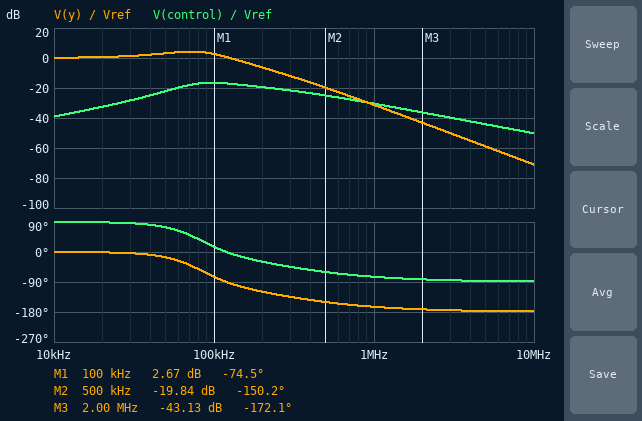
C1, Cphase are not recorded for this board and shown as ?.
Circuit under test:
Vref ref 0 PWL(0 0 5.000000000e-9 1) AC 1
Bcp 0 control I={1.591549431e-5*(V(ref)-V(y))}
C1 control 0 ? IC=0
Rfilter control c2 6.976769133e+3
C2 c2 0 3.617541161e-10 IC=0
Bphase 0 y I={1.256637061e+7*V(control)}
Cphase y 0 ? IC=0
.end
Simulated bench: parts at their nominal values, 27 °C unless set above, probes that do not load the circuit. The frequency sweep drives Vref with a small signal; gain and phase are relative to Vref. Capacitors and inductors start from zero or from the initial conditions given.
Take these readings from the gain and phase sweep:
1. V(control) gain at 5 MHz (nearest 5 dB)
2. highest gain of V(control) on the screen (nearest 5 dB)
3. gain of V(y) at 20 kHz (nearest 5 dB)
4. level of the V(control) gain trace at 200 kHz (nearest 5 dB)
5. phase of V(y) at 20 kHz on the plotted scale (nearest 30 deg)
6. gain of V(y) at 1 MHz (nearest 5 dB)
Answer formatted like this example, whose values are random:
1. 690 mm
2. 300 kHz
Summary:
1. -45 dB
2. -15 dB
3. 0 dB
4. -20 dB
5. 0 deg
6. -30 dB
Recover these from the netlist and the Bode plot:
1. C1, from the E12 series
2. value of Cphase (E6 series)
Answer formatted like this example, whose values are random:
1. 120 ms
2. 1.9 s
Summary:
1. 82 pF
2. 2.2 F
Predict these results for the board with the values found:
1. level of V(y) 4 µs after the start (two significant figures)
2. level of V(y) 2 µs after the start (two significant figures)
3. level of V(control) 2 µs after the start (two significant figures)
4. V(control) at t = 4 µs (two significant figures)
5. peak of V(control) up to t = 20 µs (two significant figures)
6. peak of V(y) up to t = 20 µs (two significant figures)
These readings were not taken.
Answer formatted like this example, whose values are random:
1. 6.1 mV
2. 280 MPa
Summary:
1. 1.3 V
2. 800 mV
3. 76 mV
4. 19 mV
5. 87 mV
6. 1.4 V
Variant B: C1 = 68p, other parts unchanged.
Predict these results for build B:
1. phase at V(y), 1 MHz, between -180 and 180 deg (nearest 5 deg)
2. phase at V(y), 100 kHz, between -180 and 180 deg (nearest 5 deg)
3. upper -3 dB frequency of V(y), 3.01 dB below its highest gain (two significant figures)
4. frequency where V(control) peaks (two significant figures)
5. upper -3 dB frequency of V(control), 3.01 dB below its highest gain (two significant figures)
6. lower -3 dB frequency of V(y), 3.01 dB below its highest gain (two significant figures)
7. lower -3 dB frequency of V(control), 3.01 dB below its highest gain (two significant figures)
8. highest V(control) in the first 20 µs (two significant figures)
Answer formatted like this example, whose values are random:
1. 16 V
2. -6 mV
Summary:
1. -160 deg
2. -70 deg
3. 120 kHz
4. 100 kHz
5. 240 kHz
6. 24 kHz
7. 61 kHz
8. 89 mV
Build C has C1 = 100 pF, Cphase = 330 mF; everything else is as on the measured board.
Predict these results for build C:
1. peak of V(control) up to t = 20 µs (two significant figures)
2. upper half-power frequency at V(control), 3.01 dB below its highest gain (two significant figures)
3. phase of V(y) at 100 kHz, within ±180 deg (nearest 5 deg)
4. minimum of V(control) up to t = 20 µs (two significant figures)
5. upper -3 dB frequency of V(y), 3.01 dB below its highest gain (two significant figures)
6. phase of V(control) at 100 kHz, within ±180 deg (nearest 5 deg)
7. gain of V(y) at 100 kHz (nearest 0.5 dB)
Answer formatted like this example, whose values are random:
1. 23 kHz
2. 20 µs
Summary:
1. 45 mV
2. 500 kHz
3. -5 deg
4. -18 mV
5. 440 kHz
6. 85 deg
7. 1.0 dB
